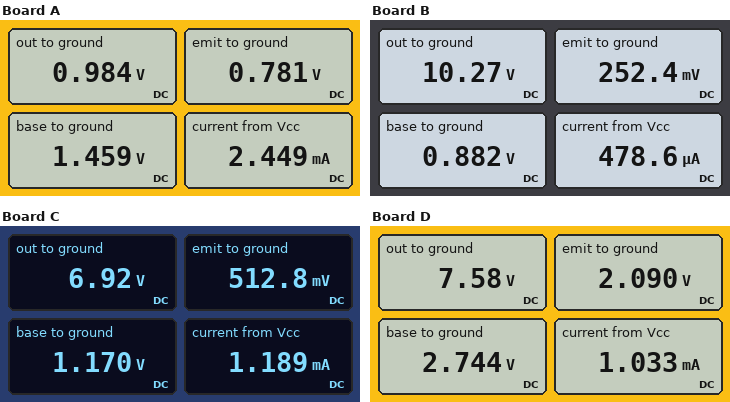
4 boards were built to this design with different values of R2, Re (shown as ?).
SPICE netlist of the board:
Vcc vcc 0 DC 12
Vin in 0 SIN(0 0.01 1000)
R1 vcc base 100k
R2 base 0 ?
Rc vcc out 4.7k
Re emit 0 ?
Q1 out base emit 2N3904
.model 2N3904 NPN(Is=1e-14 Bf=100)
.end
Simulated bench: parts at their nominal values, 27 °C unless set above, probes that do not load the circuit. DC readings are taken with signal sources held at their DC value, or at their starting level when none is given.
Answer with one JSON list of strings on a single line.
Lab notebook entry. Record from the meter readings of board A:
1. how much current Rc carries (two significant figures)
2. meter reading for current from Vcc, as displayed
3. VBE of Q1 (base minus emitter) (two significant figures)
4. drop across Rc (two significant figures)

["2.3 mA", "2.449 mA", "680 mV", "11 V"]
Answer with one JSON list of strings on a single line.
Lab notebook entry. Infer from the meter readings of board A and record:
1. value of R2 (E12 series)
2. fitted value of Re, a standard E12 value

["18 kΩ", "330 Ω"]
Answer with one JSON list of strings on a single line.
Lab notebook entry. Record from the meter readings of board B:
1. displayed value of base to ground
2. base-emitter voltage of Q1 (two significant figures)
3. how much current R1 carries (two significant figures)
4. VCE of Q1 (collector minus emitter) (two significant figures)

["0.882 V", "630 mV", "110 µA", "10 V"]
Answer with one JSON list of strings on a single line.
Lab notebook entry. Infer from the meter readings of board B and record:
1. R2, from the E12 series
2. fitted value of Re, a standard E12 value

["8.2 kΩ", "680 Ω"]
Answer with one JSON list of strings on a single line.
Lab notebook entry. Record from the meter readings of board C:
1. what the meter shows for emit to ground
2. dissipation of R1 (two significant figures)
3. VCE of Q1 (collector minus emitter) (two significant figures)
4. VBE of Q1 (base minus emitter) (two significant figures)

["512.8 mV", "1.2 mW", "6.4 V", "660 mV"]
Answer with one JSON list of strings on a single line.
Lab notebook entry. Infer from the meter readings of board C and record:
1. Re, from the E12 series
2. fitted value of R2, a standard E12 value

["470 Ω", "12 kΩ"]
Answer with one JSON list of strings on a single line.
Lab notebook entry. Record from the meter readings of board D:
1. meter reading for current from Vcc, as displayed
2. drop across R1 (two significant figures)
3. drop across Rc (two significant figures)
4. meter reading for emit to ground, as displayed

["1.033 mA", "9.3 V", "4.4 V", "2.090 V"]
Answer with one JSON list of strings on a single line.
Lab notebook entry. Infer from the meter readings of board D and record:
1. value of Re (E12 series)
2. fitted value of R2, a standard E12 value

["2.2 kΩ", "33 kΩ"]
